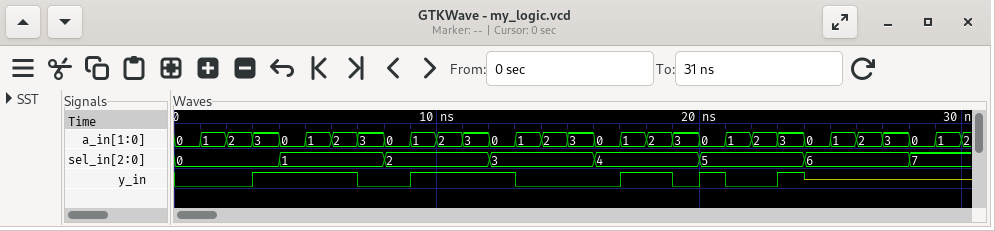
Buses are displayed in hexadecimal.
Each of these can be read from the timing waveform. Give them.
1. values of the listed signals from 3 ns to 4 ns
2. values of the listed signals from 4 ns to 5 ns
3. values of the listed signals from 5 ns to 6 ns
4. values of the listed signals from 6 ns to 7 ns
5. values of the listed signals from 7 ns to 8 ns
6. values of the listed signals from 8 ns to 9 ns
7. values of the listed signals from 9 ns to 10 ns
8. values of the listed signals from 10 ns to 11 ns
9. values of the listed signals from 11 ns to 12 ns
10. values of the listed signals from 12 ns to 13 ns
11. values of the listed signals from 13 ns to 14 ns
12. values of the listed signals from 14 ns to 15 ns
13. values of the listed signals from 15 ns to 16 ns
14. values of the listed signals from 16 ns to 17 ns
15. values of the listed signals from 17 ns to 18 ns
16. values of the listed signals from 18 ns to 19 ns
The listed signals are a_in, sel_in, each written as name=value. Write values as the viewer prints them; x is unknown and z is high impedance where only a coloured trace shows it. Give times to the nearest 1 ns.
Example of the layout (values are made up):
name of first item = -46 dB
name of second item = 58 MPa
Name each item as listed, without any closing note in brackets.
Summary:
values of the listed signals from 3 ns to 4 ns = a_in=3, sel_in=0
values of the listed signals from 4 ns to 5 ns = a_in=0, sel_in=1
values of the listed signals from 5 ns to 6 ns = a_in=1, sel_in=1
values of the listed signals from 6 ns to 7 ns = a_in=2, sel_in=1
values of the listed signals from 7 ns to 8 ns = a_in=3, sel_in=1
values of the listed signals from 8 ns to 9 ns = a_in=0, sel_in=2
values of the listed signals from 9 ns to 10 ns = a_in=1, sel_in=2
values of the listed signals from 10 ns to 11 ns = a_in=2, sel_in=2
values of the listed signals from 11 ns to 12 ns = a_in=3, sel_in=2
values of the listed signals from 12 ns to 13 ns = a_in=0, sel_in=3
values of the listed signals from 13 ns to 14 ns = a_in=1, sel_in=3
values of the listed signals from 14 ns to 15 ns = a_in=2, sel_in=3
values of the listed signals from 15 ns to 16 ns = a_in=3, sel_in=3
values of the listed signals from 16 ns to 17 ns = a_in=0, sel_in=4
values of the listed signals from 17 ns to 18 ns = a_in=1, sel_in=4
values of the listed signals from 18 ns to 19 ns = a_in=2, sel_in=4
